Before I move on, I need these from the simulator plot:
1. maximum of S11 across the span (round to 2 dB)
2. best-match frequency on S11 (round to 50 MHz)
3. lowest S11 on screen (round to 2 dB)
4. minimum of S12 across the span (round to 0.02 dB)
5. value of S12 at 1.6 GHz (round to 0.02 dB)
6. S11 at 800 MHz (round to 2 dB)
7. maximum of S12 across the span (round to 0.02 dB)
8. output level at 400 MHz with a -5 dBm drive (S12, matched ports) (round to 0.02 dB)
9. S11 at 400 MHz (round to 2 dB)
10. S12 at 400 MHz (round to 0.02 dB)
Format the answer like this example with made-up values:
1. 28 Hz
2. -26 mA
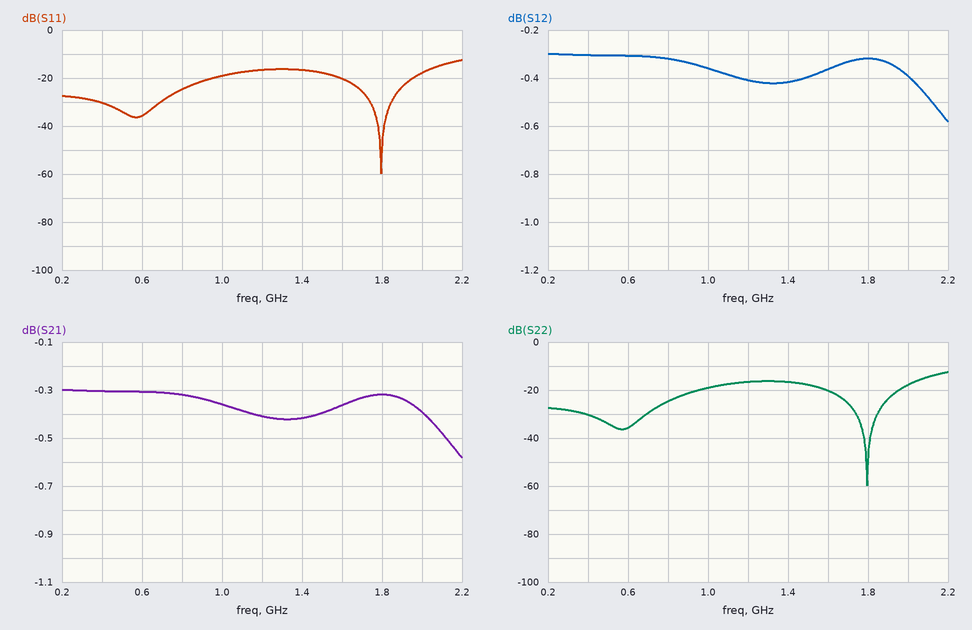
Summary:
1. -12 dB
2. 1.80 GHz
3. -60 dB
4. -0.58 dB
5. -0.36 dB
6. -24 dB
7. -0.30 dB
8. -5.30 dBm
9. -30 dB
10. -0.30 dB
